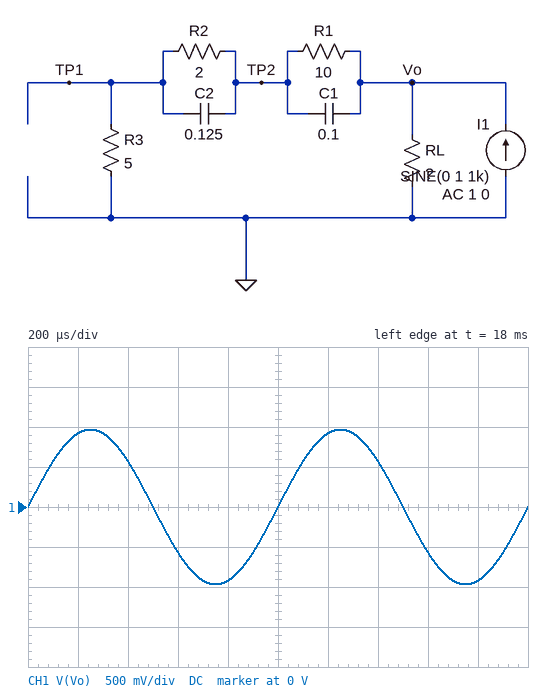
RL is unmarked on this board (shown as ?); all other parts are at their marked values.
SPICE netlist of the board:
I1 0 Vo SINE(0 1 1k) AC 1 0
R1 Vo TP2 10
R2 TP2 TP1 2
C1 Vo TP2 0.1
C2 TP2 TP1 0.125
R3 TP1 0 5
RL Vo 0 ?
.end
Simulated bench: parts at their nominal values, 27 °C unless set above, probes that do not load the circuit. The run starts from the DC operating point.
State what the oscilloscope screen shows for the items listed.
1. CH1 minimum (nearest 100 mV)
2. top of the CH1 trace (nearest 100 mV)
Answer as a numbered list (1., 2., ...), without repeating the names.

1. -1.0 V
2. 1.0 V
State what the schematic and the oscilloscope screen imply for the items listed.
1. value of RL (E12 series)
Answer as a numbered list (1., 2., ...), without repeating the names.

1. 1.2 Ω
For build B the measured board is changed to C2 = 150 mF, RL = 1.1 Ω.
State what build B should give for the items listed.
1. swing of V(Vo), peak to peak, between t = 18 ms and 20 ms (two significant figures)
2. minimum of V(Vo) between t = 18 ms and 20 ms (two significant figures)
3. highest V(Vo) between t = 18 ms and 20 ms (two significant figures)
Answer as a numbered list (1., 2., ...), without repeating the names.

1. 1.8 V
2. -900 mV
3. 900 mV
